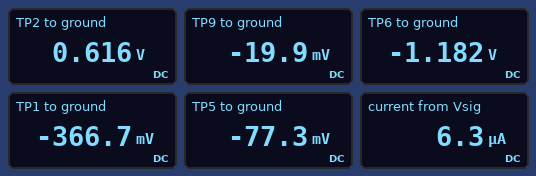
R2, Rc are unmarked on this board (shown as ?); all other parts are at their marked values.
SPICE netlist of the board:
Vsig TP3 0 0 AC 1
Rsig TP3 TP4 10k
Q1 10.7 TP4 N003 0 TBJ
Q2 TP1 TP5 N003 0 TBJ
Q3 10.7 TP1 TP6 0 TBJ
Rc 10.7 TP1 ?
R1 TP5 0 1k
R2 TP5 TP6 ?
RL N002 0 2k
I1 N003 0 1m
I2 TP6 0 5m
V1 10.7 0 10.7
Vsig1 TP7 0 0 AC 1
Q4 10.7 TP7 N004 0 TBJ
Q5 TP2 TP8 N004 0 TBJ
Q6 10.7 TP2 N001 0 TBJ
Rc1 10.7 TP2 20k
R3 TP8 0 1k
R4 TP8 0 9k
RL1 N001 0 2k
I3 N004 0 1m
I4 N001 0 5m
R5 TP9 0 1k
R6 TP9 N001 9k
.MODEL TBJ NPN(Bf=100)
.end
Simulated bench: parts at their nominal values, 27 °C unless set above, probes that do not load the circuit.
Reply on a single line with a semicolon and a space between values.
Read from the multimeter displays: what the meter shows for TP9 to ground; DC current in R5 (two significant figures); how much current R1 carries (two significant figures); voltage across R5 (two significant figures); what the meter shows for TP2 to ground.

-19.9 mV; 20 µA; 77 µA; 20 mV; 0.616 V
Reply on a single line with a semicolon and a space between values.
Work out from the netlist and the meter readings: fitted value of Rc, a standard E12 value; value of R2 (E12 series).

27 kΩ; 15 kΩ
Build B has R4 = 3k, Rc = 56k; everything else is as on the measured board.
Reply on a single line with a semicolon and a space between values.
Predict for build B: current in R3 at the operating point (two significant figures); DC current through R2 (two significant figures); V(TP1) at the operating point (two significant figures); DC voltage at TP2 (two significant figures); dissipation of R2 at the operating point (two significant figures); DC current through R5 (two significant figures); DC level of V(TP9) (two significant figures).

3.5 µA; 99 µA; -790 mV; 510 mV; 150 µW; 31 µA; -31 mV
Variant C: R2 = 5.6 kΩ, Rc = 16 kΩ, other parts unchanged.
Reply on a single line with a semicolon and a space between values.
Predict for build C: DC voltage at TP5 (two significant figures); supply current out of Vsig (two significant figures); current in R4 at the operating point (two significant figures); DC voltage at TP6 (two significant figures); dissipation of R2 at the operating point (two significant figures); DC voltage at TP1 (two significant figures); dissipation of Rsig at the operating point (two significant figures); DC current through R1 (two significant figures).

-32 mV; 4.1 µA; 460 nA; -180 mV; 3.9 µW; 640 mV; 170 nW; 32 µA
